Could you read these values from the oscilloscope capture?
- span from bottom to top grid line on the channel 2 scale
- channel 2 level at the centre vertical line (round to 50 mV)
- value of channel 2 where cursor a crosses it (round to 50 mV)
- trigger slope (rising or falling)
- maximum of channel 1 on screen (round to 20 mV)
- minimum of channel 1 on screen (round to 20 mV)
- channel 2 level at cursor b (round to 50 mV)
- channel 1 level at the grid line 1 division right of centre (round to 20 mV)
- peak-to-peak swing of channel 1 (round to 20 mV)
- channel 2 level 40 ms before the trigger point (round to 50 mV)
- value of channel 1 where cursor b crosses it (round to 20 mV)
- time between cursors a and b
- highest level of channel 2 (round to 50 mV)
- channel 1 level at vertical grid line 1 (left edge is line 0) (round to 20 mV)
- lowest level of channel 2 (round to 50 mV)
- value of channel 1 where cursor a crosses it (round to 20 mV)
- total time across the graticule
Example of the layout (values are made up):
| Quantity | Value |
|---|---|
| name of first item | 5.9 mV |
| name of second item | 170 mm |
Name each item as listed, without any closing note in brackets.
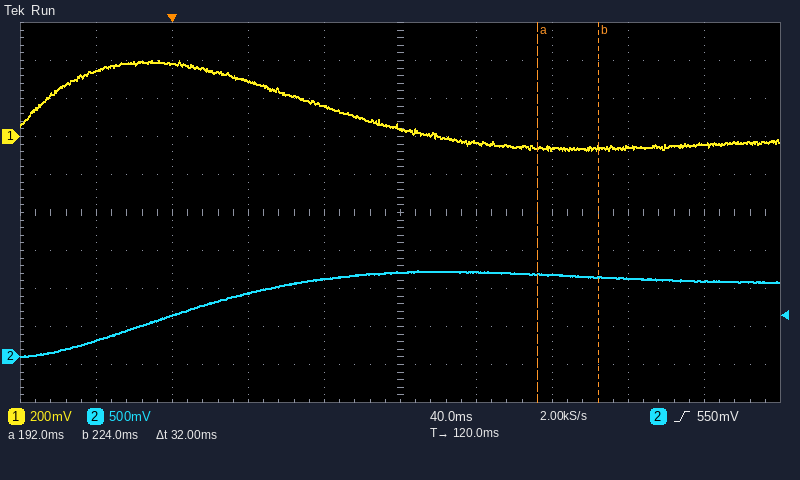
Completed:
| Quantity | Value |
|---|---|
| span from bottom to top grid line on the channel 2 scale | 5 V |
| channel 2 level at the centre vertical line | 1.10 V |
| value of channel 2 where cursor a crosses it | 1.10 V |
| trigger slope | rising |
| maximum of channel 1 on screen | 400 mV |
| minimum of channel 1 on screen | -80 mV |
| channel 2 level at cursor b | 1.05 V |
| channel 1 level at the grid line 1 division right of centre | -40 mV |
| peak-to-peak swing of channel 1 | 480 mV |
| channel 2 level 40 ms before the trigger point | 200 mV |
| value of channel 1 where cursor b crosses it | -60 mV |
| time between cursors a and b | 32 ms |
| highest level of channel 2 | 1.15 V |
| channel 1 level at vertical grid line 1 (left edge is line 0) | 340 mV |
| lowest level of channel 2 | 0 mV |
| value of channel 1 where cursor a crosses it | -60 mV |
| total time across the graticule | 400 ms |
